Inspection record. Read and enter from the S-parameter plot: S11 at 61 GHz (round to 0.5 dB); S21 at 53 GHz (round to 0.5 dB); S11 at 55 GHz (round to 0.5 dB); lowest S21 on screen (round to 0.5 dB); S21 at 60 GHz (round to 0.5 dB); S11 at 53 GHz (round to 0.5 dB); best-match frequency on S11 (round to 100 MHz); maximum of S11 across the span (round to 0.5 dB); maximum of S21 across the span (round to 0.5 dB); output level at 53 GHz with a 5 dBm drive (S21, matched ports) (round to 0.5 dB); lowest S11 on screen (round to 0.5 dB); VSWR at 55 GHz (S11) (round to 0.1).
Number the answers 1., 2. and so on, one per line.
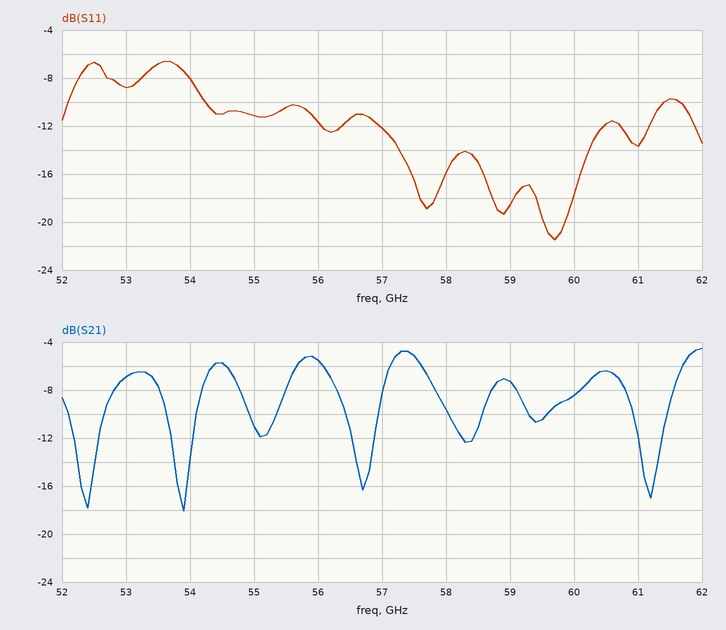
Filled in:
1. -13.5 dB
2. -7.0 dB
3. -11.0 dB
4. -18.0 dB
5. -8.5 dB
6. -9.0 dB
7. 59.7 GHz
8. -6.5 dB
9. -4.5 dB
10. -2.0 dBm
11. -21.5 dB
12. 1.8
